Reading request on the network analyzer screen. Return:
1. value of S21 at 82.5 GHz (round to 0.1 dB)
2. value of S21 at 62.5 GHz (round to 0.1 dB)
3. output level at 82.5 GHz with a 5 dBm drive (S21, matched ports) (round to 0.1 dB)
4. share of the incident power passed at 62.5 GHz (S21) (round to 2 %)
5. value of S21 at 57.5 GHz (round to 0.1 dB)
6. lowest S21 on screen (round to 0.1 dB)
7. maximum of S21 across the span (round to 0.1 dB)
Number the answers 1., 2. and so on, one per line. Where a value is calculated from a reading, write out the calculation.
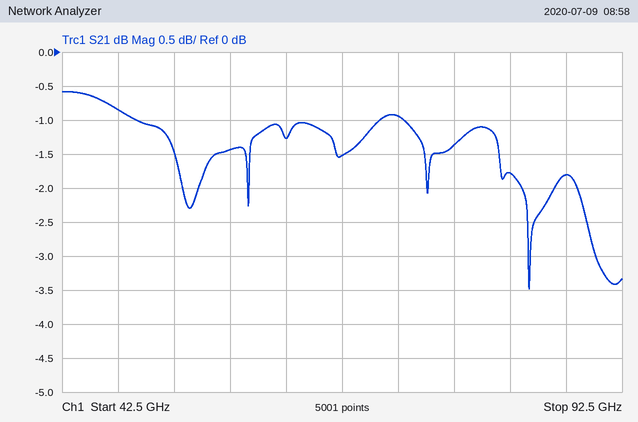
1. -1.8 dB
2. -1.3 dB
3. 5 dBm + (-1.8 dB) = 3.2 dBm
4. 10^(-1.3/10) ≈ 74 %
5. -1.4 dB
6. -3.5 dB
7. -0.6 dB
